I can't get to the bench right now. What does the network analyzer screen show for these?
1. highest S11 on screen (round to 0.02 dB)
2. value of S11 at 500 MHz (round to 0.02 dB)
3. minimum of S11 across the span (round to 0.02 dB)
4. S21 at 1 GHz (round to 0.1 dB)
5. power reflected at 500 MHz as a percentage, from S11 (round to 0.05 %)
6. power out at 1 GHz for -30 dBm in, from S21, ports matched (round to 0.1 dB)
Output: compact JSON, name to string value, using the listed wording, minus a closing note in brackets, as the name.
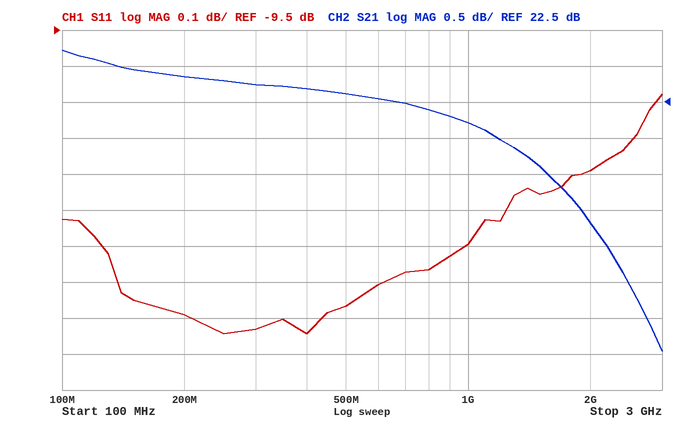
{"highest S11 on screen": "-9.68 dB", "value of S11 at 500 MHz": "-10.26 dB", "minimum of S11 across the span": "-10.34 dB", "S21 at 1 GHz": "22.2 dB", "power reflected at 500 MHz as a percentage, from S11": "9.40 %", "power out at 1 GHz for -30 dBm in, from S21, ports matched": "-7.8 dBm"}
